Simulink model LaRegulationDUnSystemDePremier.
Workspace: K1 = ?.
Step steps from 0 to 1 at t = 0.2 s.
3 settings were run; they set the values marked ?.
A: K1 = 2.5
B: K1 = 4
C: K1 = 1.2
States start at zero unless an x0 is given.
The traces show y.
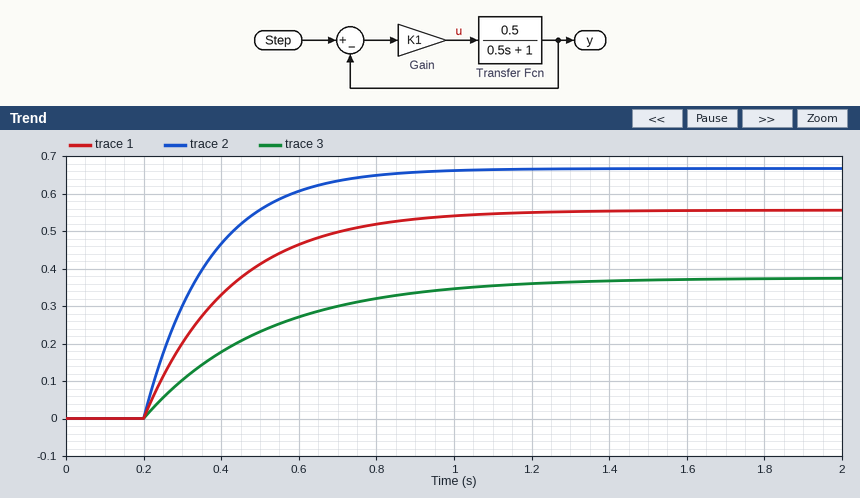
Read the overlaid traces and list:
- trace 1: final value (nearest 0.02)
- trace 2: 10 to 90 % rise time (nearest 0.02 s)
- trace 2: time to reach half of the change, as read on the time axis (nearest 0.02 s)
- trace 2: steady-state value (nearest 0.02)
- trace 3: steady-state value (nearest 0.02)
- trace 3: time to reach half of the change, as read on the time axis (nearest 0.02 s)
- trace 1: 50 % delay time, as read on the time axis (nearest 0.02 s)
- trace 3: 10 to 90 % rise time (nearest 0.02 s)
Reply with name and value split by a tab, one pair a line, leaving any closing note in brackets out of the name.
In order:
trace 1: final value	0.56
trace 2: 10 to 90 % rise time	0.36 s
trace 2: time to reach half of the change, as read on the time axis	0.32 s
trace 2: steady-state value	0.66
trace 3: steady-state value	0.38
trace 3: time to reach half of the change, as read on the time axis	0.42 s
trace 1: 50 % delay time, as read on the time axis	0.36 s
trace 3: 10 to 90 % rise time	0.68 s
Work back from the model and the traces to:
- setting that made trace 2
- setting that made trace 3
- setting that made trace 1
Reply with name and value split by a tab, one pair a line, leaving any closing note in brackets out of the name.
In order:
setting that made trace 2	B
setting that made trace 3	C
setting that made trace 1	A
